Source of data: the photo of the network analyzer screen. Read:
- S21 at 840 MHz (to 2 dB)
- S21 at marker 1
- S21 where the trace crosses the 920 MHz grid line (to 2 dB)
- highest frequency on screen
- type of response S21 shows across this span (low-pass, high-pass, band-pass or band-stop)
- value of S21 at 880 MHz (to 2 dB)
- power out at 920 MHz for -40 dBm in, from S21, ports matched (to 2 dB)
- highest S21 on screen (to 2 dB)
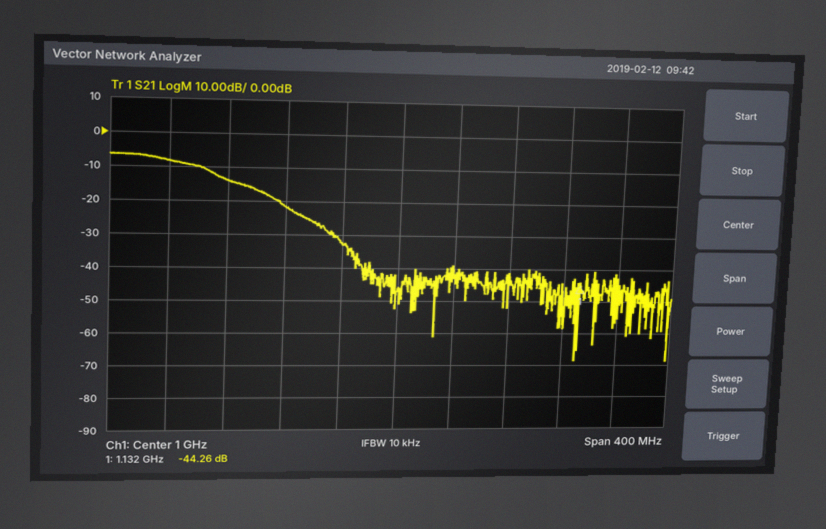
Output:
-8 dB
-44.26 dB
-22 dB
1.2 GHz
low-pass
-14 dB
-62 dBm
-6 dB
